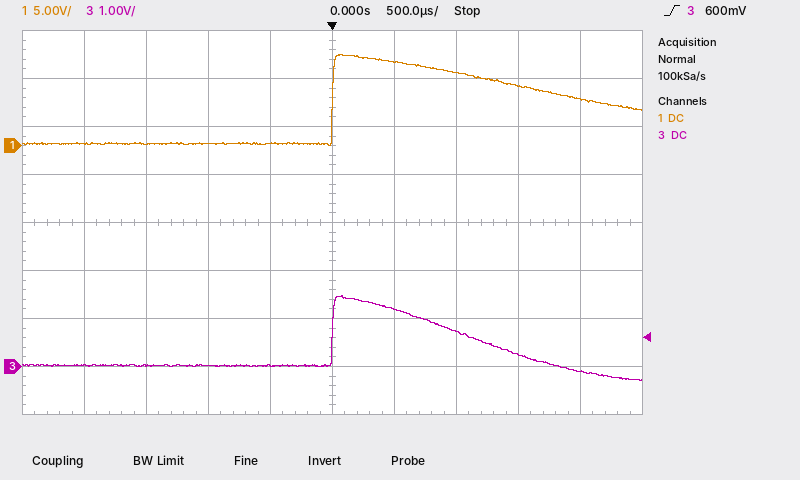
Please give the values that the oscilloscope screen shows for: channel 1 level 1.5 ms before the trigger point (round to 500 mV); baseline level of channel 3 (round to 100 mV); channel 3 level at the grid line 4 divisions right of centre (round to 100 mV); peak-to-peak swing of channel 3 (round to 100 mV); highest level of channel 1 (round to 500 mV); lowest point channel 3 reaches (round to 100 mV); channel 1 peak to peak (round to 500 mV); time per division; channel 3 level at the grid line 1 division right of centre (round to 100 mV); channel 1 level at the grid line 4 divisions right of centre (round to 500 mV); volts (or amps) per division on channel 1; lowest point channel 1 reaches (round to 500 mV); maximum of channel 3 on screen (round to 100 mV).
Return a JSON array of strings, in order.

["0.0 V", "0.0 V", "-100 mV", "1.8 V", "9.5 V", "-300 mV", "9.5 V", "500 µs", "1.2 V", "5.0 V", "5 V", "0.0 V", "1.5 V"]
